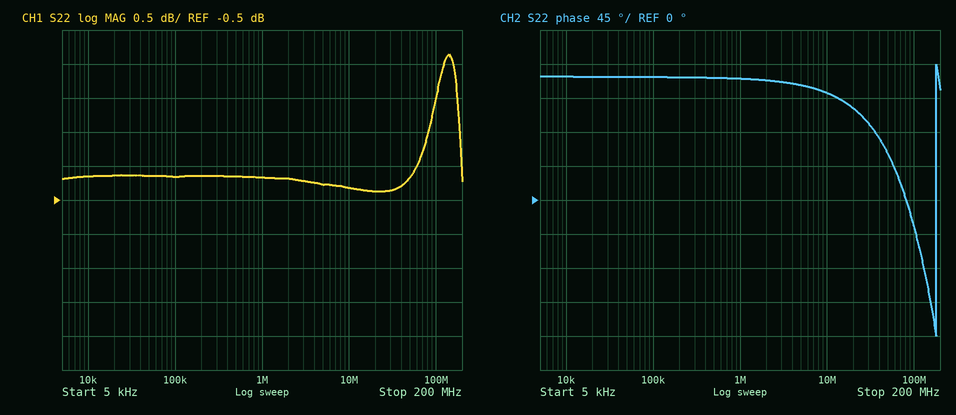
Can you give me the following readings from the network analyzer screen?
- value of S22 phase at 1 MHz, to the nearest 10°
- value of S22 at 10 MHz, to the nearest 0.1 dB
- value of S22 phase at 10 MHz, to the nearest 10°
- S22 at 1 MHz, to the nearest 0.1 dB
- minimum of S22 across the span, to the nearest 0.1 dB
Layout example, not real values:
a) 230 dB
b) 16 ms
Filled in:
a) 160°
b) -0.3 dB
c) 140°
d) -0.2 dB
e) -0.4 dB
